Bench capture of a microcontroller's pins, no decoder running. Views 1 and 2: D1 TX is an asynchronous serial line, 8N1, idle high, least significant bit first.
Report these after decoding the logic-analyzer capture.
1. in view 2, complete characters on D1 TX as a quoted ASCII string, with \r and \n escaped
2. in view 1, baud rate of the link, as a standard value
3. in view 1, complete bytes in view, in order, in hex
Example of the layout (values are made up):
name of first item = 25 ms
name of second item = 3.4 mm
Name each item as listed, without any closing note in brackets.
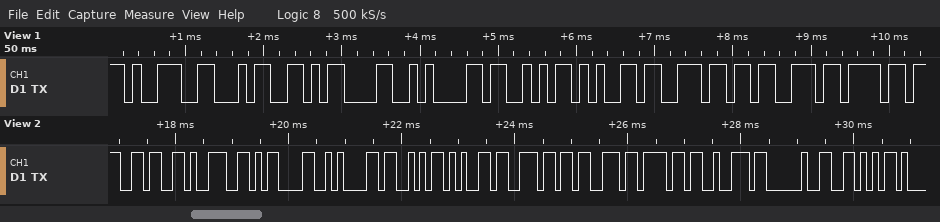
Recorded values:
in view 2, complete characters on D1 TX as a quoted ASCII string, with \r and \n escaped = "69\r\nSensor V"
in view 1, baud rate of the link, as a standard value = 9600 baud
in view 1, complete bytes in view, in order, in hex = 0x39 0x34 0x0D 0x0A 0x53 0x65 0x6E 0x73 0x6F
